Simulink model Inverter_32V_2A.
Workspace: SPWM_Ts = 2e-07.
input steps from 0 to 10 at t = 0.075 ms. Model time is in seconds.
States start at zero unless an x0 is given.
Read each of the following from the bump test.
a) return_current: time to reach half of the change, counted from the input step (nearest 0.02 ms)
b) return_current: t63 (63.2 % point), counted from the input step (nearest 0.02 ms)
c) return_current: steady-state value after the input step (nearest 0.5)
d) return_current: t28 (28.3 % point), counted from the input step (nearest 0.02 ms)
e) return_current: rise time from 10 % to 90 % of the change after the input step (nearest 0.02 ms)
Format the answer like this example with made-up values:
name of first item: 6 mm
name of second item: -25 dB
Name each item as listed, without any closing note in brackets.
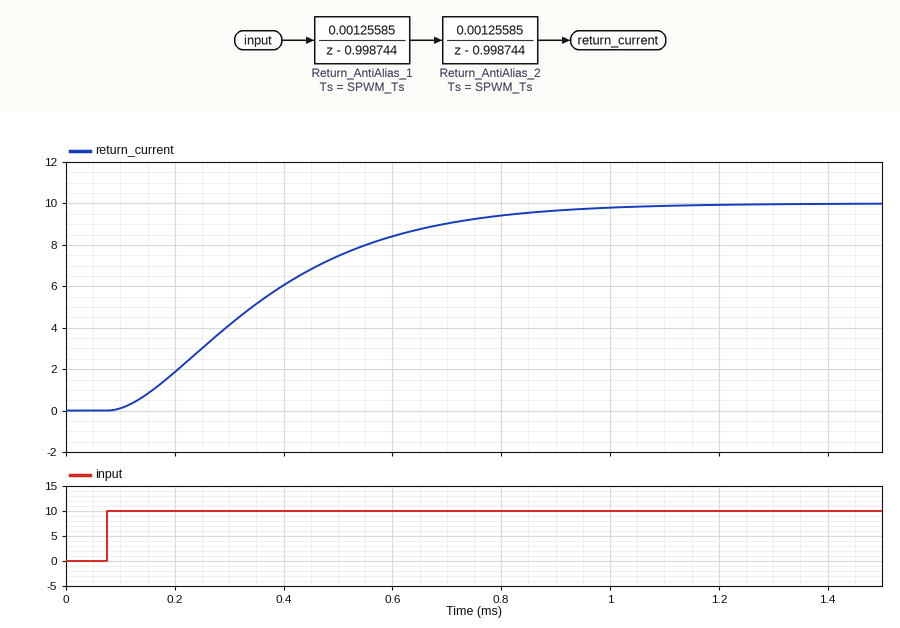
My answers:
return_current: time to reach half of the change, counted from the input step: 0.26 ms
return_current: t63 (63.2 % point), counted from the input step: 0.34 ms
return_current: steady-state value after the input step: 10.0
return_current: t28 (28.3 % point), counted from the input step: 0.16 ms
return_current: rise time from 10 % to 90 % of the change after the input step: 0.54 ms
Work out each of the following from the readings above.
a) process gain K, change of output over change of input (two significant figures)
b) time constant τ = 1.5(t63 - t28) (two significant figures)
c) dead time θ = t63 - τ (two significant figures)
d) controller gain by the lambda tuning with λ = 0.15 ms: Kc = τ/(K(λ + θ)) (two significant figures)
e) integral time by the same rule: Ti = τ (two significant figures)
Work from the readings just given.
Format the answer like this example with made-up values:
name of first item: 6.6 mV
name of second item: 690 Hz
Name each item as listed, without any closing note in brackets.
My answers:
process gain K, change of output over change of input: 1.0
time constant τ = 1.5(t63 - t28): 0.27 ms
dead time θ = t63 - τ: 0.070 ms
controller gain by the lambda tuning with λ = 0.15 ms: Kc = τ/(K(λ + θ)): 1.2
integral time by the same rule: Ti = τ: 0.27 ms
